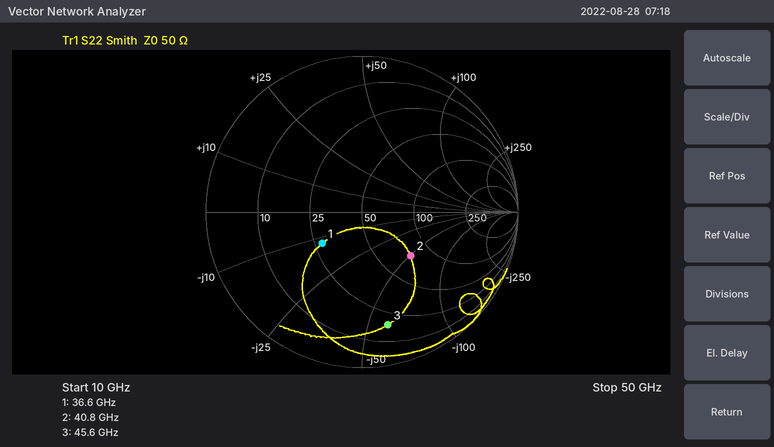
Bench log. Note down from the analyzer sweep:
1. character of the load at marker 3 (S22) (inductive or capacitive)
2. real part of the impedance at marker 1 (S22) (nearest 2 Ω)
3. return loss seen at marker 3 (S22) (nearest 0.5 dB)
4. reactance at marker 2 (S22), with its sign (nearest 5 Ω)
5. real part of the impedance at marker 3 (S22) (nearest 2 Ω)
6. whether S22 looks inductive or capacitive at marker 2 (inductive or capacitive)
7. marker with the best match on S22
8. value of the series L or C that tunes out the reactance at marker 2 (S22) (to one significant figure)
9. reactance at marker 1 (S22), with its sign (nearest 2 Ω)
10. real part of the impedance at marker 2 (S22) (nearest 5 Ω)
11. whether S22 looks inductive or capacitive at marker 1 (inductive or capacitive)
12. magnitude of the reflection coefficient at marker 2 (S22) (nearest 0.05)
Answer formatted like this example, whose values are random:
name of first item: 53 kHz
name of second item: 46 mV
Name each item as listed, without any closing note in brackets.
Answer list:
character of the load at marker 3 (S22): capacitive
real part of the impedance at marker 1 (S22): 28 Ω
return loss seen at marker 3 (S22): 2.5 dB
reactance at marker 2 (S22), with its sign: -50 Ω
real part of the impedance at marker 3 (S22): 18 Ω
whether S22 looks inductive or capacitive at marker 2: capacitive
marker with the best match on S22: marker 1
value of the series L or C that tunes out the reactance at marker 2 (S22): 200 pH
reactance at marker 1 (S22), with its sign: -12 Ω
real part of the impedance at marker 2 (S22): 75 Ω
whether S22 looks inductive or capacitive at marker 1: capacitive
magnitude of the reflection coefficient at marker 2 (S22): 0.40
